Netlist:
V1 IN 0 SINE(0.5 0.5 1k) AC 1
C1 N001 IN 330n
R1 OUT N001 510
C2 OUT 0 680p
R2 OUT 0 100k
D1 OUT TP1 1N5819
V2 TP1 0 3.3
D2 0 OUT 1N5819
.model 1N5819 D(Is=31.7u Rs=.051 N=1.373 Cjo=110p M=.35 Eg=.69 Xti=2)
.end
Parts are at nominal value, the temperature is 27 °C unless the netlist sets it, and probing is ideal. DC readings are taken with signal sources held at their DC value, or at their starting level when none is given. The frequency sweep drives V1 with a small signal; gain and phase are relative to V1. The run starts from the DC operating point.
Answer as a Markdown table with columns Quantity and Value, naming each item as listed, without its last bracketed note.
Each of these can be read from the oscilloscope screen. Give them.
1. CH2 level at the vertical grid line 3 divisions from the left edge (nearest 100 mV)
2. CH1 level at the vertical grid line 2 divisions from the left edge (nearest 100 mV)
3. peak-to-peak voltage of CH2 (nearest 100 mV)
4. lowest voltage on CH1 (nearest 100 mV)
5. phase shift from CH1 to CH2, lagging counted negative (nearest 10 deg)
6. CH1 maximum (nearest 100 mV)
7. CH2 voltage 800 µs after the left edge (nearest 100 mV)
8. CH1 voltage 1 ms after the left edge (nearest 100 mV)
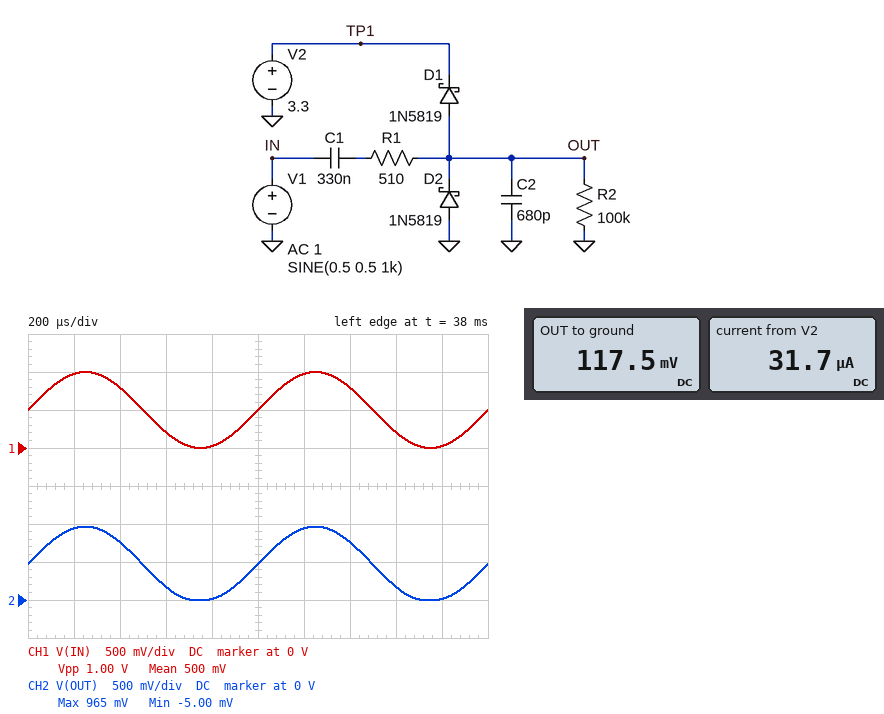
| Quantity | Value |
|---|---|
| CH2 level at the vertical grid line 3 divisions from the left edge | 200 mV |
| CH1 level at the vertical grid line 2 divisions from the left edge | 800 mV |
| peak-to-peak voltage of CH2 | 1.0 V |
| lowest voltage on CH1 | 0 V |
| phase shift from CH1 to CH2, lagging counted negative | 0 deg |
| CH1 maximum | 1.0 V |
| CH2 voltage 800 µs after the left edge | 0 V |
| CH1 voltage 1 ms after the left edge | 500 mV |
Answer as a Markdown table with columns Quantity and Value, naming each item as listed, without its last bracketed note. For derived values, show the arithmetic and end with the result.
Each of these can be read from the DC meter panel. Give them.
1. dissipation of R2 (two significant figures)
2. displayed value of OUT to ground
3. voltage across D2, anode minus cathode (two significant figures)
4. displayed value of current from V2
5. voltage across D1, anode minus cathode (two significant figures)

| Quantity | Value |
|---|---|
| dissipation of R2 | (117.5 mV)^2 / 100 kΩ = 140 nW |
| displayed value of OUT to ground | 117.5 mV |
| voltage across D2, anode minus cathode | 0 V - 117.5 mV = -120 mV |
| displayed value of current from V2 | 31.7 µA |
| voltage across D1, anode minus cathode | 117.5 mV - 3.3 V = -3.2 V |
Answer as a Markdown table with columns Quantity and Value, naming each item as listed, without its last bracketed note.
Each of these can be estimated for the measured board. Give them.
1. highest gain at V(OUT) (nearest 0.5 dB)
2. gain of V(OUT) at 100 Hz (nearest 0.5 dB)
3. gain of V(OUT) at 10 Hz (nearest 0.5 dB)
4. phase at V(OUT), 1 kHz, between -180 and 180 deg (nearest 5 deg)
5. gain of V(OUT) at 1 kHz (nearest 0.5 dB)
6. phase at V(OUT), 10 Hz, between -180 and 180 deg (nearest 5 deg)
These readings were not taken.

| Quantity | Value |
|---|---|
| highest gain at V(OUT) | 0 dB |
| gain of V(OUT) at 100 Hz | -0.5 dB |
| gain of V(OUT) at 10 Hz | -7.0 dB |
| phase at V(OUT), 1 kHz, between -180 and 180 deg | 0 deg |
| gain of V(OUT) at 1 kHz | 0 dB |
| phase at V(OUT), 10 Hz, between -180 and 180 deg | 60 deg |
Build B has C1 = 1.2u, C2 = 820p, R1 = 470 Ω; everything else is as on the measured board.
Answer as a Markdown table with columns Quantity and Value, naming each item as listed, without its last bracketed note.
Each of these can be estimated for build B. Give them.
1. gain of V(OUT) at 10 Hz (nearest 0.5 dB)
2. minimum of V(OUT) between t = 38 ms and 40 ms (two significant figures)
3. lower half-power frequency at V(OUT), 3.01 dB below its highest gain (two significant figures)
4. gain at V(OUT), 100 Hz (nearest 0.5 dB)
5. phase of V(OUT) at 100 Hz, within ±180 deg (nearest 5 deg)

| Quantity | Value |
|---|---|
| gain of V(OUT) at 10 Hz | -1.0 dB |
| minimum of V(OUT) between t = 38 ms and 40 ms | -8.9 mV |
| lower half-power frequency at V(OUT), 3.01 dB below its highest gain | 5.2 Hz |
| gain at V(OUT), 100 Hz | 0 dB |
| phase of V(OUT) at 100 Hz, within ±180 deg | 5 deg |
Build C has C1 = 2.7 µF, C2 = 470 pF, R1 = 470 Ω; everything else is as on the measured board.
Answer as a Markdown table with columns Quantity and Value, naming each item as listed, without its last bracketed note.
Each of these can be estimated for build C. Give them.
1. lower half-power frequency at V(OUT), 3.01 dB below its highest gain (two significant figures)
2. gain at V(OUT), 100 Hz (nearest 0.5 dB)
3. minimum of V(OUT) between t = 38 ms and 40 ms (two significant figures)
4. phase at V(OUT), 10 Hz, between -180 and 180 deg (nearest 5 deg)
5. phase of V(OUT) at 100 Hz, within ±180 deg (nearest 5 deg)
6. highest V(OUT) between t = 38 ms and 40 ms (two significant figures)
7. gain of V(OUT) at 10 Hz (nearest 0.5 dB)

| Quantity | Value |
|---|---|
| lower half-power frequency at V(OUT), 3.01 dB below its highest gain | 2.3 Hz |
| gain at V(OUT), 100 Hz | 0 dB |
| minimum of V(OUT) between t = 38 ms and 40 ms | -21 mV |
| phase at V(OUT), 10 Hz, between -180 and 180 deg | 15 deg |
| phase of V(OUT) at 100 Hz, within ±180 deg | 0 deg |
| highest V(OUT) between t = 38 ms and 40 ms | 950 mV |
| gain of V(OUT) at 10 Hz | -0.5 dB |
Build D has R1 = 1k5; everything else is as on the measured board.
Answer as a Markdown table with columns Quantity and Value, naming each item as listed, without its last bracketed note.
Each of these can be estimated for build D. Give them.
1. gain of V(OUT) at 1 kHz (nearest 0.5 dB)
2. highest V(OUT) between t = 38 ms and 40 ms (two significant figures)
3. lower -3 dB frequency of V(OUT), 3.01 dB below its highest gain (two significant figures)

| Quantity | Value |
|---|---|
| gain of V(OUT) at 1 kHz | -0.5 dB |
| highest V(OUT) between t = 38 ms and 40 ms | 940 mV |
| lower -3 dB frequency of V(OUT), 3.01 dB below its highest gain | 18 Hz |
